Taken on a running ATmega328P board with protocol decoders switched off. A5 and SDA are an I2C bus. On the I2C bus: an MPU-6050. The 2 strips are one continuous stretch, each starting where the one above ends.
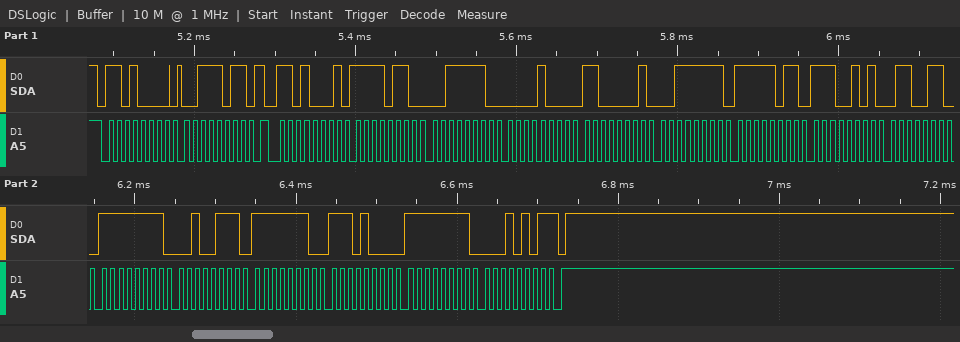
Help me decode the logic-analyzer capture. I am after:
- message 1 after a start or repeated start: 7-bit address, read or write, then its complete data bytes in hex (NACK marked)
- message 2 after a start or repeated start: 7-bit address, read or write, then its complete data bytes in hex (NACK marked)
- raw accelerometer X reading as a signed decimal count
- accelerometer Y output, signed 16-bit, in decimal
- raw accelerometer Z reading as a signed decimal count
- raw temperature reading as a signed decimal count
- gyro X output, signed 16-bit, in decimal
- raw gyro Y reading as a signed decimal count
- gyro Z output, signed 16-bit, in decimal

0x68 write: 3B
0x68 read: F6 3E 08 C1 3F FB E5 66 FF 27 FE E8 FF 15 NACK
-2498
2241
16379
-6810
-217
-280
-235
